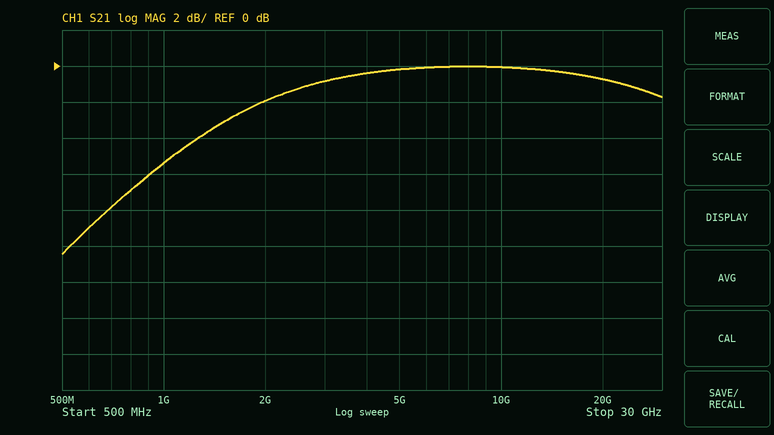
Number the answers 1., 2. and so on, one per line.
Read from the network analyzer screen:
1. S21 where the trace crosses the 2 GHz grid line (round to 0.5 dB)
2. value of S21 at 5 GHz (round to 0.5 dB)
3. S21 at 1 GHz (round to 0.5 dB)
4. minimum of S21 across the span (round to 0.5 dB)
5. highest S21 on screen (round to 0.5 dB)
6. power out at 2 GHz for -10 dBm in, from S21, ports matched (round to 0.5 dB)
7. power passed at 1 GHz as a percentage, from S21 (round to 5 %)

1. -2.0 dB
2. 0.0 dB
3. -5.5 dB
4. -10.5 dB
5. 0.0 dB
6. -12.0 dBm
7. 30 %
